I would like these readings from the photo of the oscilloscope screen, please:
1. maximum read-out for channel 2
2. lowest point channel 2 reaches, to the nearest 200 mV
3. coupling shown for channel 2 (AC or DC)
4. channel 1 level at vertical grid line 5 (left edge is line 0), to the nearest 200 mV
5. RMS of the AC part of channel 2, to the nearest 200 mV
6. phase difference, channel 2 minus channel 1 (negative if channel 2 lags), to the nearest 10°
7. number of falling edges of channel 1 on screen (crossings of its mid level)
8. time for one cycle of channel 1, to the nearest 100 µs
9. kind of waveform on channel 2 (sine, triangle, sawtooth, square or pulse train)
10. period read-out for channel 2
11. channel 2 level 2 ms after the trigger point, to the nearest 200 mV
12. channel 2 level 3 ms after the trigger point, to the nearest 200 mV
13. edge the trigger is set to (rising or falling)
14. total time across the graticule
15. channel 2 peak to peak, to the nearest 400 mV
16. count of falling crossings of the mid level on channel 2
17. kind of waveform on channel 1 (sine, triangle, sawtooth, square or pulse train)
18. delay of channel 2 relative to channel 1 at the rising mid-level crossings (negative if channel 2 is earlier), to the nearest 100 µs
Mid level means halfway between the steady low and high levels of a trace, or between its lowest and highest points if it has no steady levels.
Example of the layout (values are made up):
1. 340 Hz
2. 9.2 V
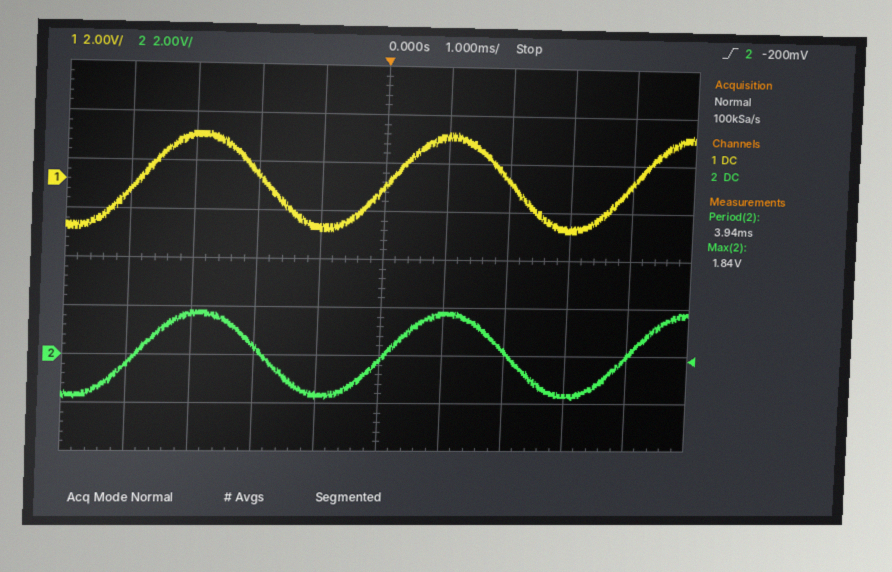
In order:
1. 1.84 V
2. -1.8 V
3. DC
4. -200 mV
5. 1.2 V
6. 0°
7. 2
8. 3.9 ms
9. sine
10. 3.94 ms
11. 200 mV
12. -1.6 V
13. rising
14. 10 ms
15. 3.6 V
16. 2
17. sine
18. 0.0 ms
